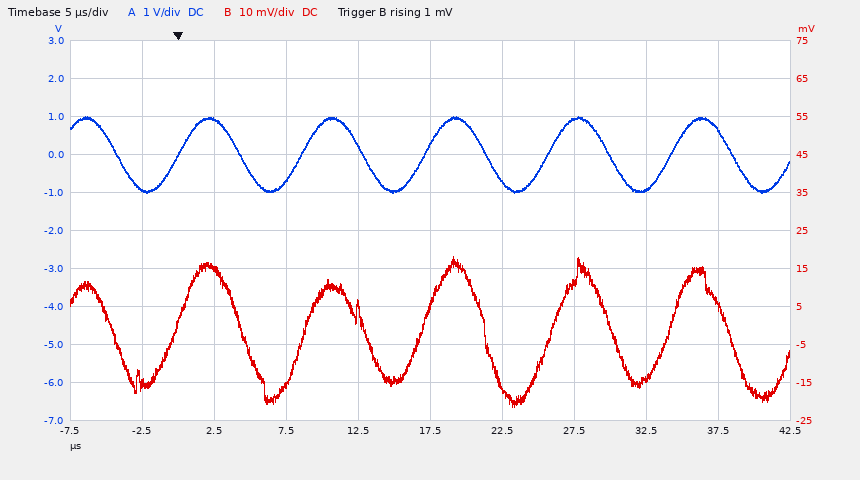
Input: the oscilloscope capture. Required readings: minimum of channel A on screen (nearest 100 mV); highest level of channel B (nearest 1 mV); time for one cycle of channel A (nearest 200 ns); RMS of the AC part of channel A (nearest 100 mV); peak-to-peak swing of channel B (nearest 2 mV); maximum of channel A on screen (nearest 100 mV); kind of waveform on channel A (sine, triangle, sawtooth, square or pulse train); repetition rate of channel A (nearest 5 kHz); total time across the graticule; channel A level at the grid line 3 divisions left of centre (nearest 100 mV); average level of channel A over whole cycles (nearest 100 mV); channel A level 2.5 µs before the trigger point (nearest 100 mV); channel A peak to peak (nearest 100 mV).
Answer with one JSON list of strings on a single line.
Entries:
["-1.0 V", "18 mV", "8.6 µs", "700 mV", "40 mV", "1.0 V", "sine", "115 kHz", "50 µs", "900 mV", "0.0 V", "-900 mV", "2.0 V"]
